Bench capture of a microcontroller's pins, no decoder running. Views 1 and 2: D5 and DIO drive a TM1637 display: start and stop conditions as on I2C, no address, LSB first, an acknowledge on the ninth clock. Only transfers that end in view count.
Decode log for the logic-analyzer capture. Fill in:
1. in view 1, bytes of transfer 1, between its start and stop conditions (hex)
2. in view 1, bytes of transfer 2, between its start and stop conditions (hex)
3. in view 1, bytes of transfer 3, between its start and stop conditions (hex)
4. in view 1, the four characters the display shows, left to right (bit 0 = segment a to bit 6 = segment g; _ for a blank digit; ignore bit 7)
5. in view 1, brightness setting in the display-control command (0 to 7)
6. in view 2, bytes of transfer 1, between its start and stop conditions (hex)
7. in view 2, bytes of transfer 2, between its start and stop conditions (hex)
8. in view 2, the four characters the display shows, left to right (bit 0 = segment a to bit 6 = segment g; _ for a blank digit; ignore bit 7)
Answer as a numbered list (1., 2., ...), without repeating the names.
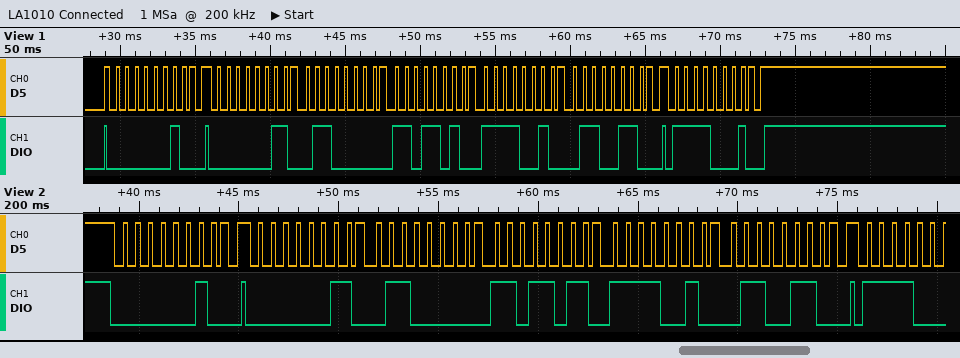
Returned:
1. 40
2. C0 06 5B 4F 66
3. 8F
4. 1234
5. 7
6. 40
7. C0 06 DB 4F 66
8. 1234
